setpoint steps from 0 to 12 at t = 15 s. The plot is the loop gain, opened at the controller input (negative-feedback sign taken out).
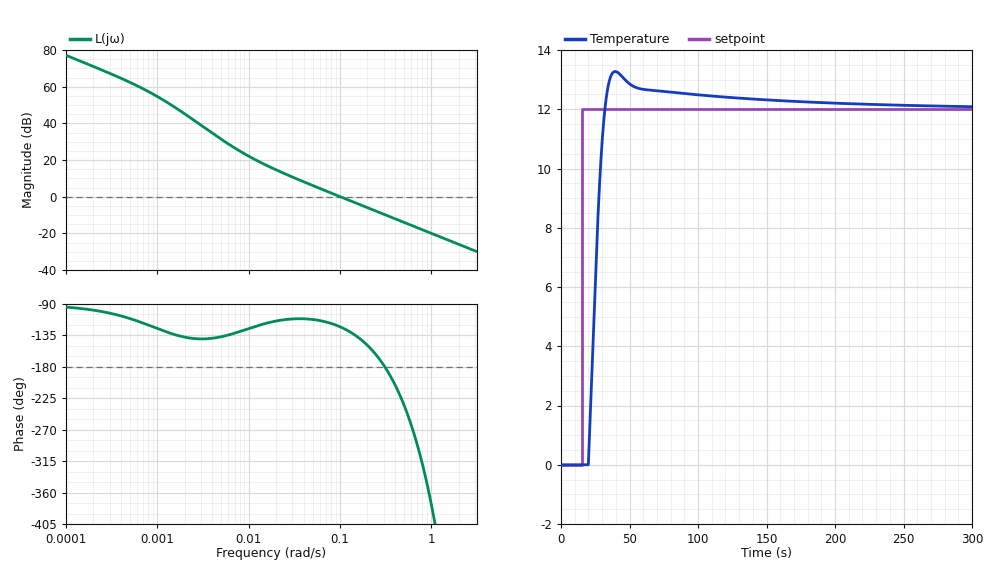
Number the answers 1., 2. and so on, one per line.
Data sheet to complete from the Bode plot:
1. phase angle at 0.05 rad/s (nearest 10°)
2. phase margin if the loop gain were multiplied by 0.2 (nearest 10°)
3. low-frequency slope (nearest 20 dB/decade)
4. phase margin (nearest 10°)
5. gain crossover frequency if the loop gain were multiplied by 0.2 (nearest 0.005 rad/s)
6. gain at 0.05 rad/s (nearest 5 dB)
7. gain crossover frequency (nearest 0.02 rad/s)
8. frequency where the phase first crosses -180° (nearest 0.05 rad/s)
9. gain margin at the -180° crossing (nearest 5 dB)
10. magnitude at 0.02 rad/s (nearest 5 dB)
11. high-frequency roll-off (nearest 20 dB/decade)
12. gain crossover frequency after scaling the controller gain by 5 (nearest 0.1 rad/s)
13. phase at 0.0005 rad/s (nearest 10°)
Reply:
1. -110°
2. 70°
3. -20 dB/decade
4. 60°
5. 0.020 rad/s
6. 5 dB
7. 0.10 rad/s
8. 0.30 rad/s
9. 10 dB
10. 15 dB
11. -20 dB/decade
12. 0.5 rad/s
13. -110°
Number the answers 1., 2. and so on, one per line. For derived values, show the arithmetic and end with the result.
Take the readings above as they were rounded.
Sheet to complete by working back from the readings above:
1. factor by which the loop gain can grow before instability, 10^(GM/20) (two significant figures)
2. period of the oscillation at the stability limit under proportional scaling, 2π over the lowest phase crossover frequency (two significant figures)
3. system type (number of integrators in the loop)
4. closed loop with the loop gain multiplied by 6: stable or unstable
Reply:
1. 10^(10 / 20) = 3.2
2. 2π / 0.3 = 21 s
3. 1
4. unstable
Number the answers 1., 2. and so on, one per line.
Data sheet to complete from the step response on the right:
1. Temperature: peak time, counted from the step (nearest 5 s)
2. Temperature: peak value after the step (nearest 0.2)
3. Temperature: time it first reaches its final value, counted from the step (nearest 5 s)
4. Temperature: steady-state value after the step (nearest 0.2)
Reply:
1. 25 s
2. 13.2
3. 15 s
4. 12.0
